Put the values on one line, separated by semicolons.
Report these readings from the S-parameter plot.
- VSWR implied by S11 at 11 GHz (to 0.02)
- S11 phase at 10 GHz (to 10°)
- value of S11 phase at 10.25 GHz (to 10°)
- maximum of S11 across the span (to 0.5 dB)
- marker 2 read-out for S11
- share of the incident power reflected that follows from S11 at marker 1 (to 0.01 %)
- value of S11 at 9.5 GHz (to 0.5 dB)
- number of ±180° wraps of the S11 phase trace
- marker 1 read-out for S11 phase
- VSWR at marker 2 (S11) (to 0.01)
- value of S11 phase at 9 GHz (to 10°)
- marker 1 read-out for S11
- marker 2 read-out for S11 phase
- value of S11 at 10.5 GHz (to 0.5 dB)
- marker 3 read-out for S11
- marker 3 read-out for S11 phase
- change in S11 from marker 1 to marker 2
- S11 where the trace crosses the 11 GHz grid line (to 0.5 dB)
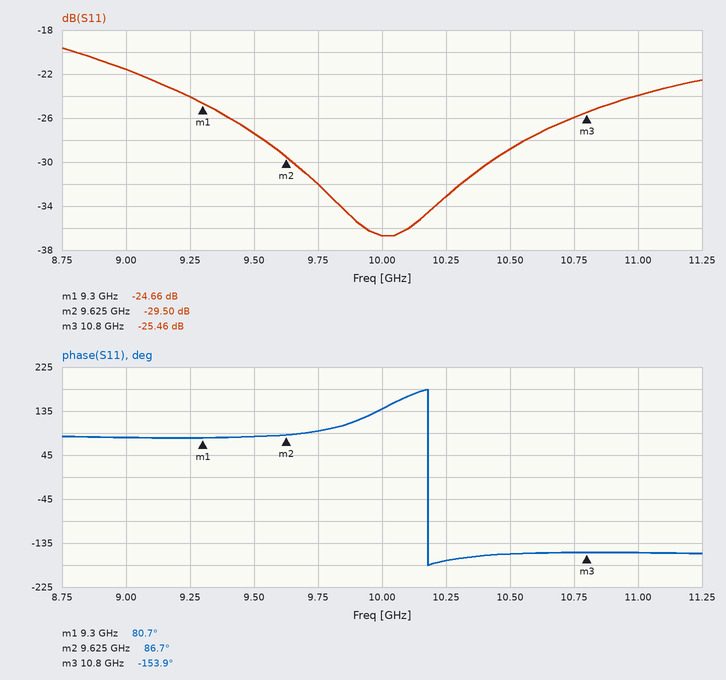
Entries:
1.14; 140°; -170°; -19.5 dB; -29.50 dB; 0.34 %; -27.5 dB; 1; 80.7°; 1.07; 80°; -24.66 dB; 86.7°; -29.0 dB; -25.46 dB; -153.9°; -4.84 dB; -24.0 dB
